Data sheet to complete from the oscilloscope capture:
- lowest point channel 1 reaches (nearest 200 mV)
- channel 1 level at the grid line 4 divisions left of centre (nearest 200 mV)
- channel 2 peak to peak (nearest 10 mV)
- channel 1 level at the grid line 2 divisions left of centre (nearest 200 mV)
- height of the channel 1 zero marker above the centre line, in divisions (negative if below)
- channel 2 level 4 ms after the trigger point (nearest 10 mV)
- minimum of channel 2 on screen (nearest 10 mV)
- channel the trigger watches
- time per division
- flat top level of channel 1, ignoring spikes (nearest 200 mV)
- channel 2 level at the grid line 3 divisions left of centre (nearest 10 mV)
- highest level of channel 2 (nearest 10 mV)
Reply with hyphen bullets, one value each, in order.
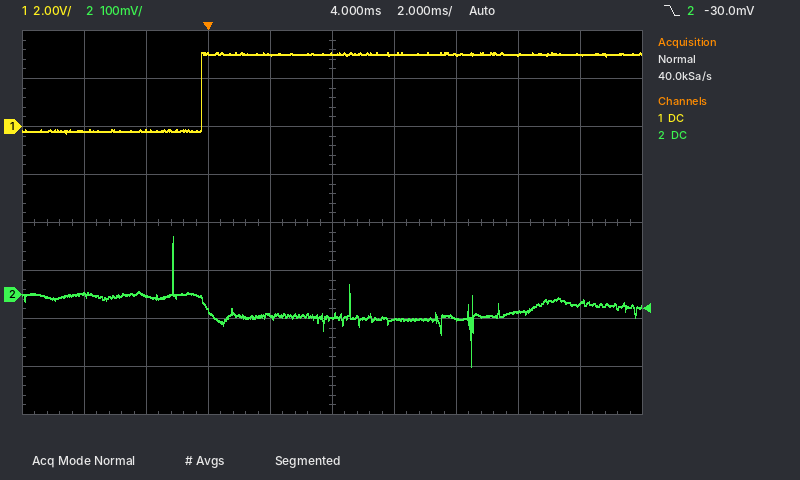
- -200 mV
- -200 mV
- 270 mV
- 3.0 V
- +2.0 div
- -50 mV
- -150 mV
- channel 2
- 2 ms
- 3.0 V
- 0 mV
- 120 mV
